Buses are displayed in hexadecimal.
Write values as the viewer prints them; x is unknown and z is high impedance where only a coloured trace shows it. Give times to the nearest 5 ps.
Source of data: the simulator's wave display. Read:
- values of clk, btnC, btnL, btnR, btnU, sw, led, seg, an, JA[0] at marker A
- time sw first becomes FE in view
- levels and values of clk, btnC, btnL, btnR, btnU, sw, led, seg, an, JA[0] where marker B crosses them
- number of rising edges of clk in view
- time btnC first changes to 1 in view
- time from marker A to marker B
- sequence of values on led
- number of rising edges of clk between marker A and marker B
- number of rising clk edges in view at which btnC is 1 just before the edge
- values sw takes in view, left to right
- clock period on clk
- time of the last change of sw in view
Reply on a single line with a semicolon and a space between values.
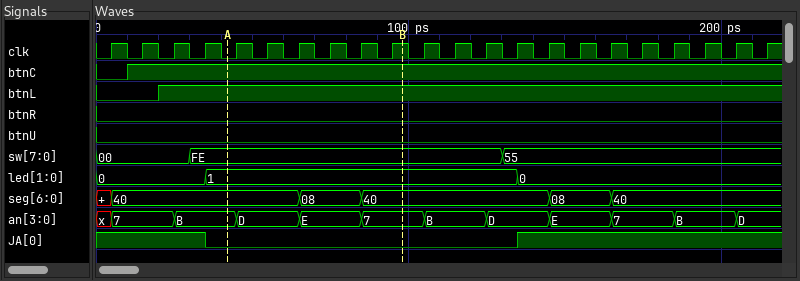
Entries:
clk=0, btnC=1, btnL=1, btnR=0, btnU=0, sw=FE, led=1, seg=40, an=B, JA[0]=0; 30 ps; clk=1, btnC=1, btnL=1, btnR=0, btnU=0, sw=FE, led=1, seg=40, an=7, JA[0]=0; 22; 10 ps; 55 ps; 0, 1, 0; 6; 21; 00, FE, 55; 10 ps; 130 ps
